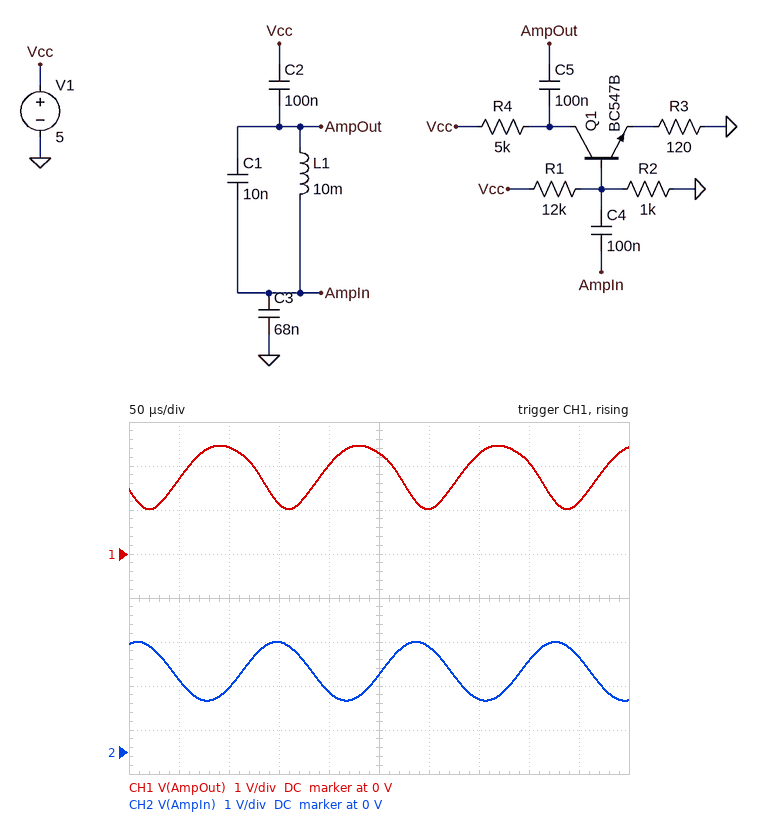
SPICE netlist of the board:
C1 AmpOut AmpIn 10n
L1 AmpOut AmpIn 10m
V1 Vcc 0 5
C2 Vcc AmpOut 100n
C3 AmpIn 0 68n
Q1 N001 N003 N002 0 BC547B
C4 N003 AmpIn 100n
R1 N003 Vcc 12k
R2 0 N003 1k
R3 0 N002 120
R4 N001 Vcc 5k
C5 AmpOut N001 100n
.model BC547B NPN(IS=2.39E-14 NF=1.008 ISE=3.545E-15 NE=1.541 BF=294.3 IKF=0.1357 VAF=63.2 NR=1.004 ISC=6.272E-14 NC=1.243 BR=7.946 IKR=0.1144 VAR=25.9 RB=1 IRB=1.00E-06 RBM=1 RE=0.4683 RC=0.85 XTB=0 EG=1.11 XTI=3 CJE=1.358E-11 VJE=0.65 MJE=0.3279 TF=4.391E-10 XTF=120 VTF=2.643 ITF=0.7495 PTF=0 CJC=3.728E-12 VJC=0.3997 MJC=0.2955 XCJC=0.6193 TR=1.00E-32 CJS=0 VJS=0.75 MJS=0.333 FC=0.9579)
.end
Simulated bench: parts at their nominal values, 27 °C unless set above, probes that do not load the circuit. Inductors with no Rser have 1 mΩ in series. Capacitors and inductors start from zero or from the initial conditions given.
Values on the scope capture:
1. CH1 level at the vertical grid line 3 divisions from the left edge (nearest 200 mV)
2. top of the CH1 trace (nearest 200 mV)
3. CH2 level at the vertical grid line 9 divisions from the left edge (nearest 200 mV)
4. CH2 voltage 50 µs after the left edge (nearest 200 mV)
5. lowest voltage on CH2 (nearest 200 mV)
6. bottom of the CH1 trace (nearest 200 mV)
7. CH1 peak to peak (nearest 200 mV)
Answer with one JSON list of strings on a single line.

["1.2 V", "2.4 V", "2.2 V", "1.6 V", "1.2 V", "1.0 V", "1.4 V"]
